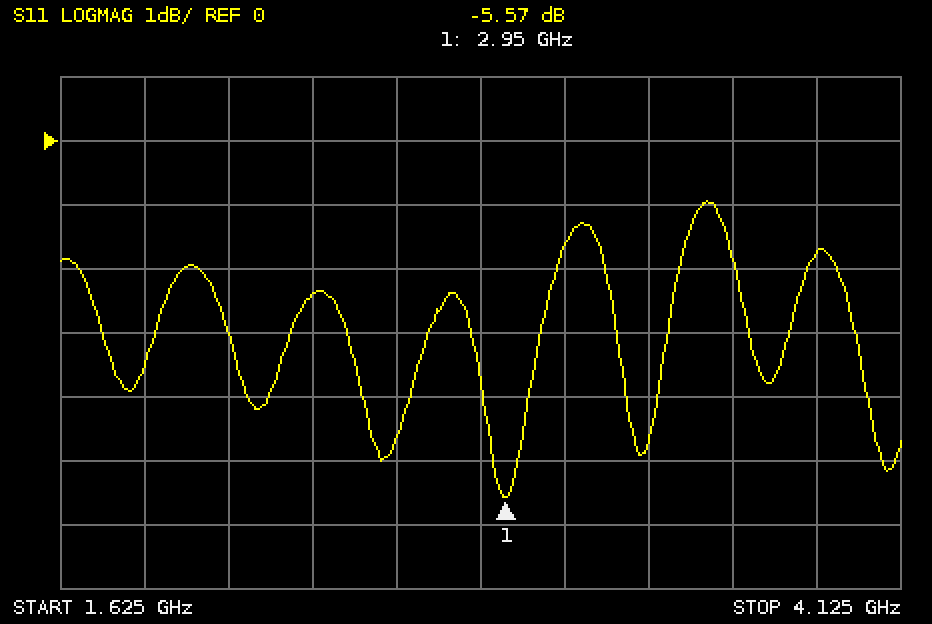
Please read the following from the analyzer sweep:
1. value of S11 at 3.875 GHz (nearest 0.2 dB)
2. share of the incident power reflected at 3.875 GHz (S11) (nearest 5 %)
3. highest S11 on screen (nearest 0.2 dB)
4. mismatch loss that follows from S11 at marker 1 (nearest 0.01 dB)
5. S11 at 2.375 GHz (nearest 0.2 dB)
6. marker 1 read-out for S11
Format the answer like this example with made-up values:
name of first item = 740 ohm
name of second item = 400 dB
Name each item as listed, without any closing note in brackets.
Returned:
value of S11 at 3.875 GHz = -1.8 dB
share of the incident power reflected at 3.875 GHz (S11) = 65 %
highest S11 on screen = -1.0 dB
mismatch loss that follows from S11 at marker 1 = 1.41 dB
S11 at 2.375 GHz = -2.4 dB
marker 1 read-out for S11 = -5.57 dB
